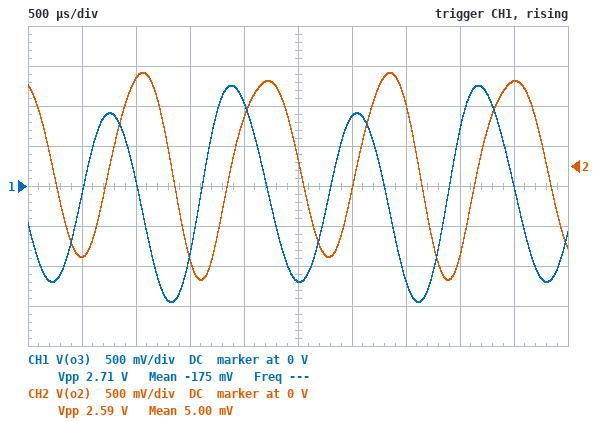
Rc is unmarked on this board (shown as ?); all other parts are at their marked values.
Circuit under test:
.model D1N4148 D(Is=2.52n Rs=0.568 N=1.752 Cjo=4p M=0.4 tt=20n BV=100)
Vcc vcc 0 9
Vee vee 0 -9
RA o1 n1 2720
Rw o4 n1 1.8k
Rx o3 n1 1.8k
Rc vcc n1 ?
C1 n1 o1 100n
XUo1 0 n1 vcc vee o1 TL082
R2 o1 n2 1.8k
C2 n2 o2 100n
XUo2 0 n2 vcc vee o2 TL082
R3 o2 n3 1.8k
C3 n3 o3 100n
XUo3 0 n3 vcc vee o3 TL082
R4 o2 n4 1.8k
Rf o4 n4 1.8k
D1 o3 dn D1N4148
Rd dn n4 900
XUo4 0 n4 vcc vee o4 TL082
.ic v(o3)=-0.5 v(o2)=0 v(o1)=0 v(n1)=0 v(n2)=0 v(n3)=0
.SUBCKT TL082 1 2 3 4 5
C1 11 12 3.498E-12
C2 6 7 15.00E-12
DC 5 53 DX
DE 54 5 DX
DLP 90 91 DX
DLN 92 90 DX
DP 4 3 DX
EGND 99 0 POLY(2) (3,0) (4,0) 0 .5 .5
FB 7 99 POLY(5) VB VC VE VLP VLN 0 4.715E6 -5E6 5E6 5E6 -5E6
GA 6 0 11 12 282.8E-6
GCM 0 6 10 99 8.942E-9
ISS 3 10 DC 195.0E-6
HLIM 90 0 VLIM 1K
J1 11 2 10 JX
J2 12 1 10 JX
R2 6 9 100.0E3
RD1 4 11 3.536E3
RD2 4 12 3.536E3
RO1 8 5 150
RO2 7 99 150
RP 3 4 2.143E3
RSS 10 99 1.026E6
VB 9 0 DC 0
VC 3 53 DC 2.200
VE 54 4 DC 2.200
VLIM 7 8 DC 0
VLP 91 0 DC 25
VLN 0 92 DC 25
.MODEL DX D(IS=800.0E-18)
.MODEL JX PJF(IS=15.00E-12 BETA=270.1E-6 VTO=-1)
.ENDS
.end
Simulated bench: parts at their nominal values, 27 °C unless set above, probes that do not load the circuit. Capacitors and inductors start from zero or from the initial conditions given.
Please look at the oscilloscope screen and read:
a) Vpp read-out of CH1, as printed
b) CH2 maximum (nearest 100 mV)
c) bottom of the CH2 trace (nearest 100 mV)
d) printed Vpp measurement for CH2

2.71 V
1.2 V
-1.4 V
2.59 V
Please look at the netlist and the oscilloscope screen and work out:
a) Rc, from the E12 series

47 kΩ
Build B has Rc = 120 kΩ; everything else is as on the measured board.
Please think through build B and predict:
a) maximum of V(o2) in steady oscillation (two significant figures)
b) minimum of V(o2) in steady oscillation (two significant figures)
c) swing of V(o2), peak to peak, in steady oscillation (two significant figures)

850 mV
-980 mV
1.8 V
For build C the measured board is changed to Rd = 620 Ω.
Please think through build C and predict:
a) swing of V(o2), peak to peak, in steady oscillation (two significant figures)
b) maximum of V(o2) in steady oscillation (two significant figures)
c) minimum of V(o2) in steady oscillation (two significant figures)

2.5 V
1.1 V
-1.4 V
